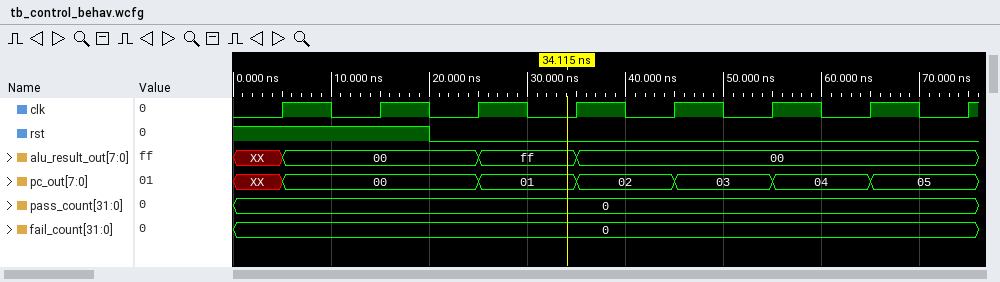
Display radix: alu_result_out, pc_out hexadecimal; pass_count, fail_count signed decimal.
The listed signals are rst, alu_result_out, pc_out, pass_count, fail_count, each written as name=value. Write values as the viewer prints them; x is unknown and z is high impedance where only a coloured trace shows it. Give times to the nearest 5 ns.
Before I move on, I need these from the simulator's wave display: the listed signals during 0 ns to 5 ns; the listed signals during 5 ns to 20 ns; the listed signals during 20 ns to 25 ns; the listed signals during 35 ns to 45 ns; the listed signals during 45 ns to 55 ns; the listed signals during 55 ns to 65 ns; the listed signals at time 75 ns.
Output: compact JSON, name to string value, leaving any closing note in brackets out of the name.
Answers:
{"the listed signals during 0 ns to 5 ns": "rst=1, alu_result_out=XX, pc_out=XX, pass_count=0, fail_count=0", "the listed signals during 5 ns to 20 ns": "rst=1, alu_result_out=00, pc_out=00, pass_count=0, fail_count=0", "the listed signals during 20 ns to 25 ns": "rst=0, alu_result_out=00, pc_out=00, pass_count=0, fail_count=0", "the listed signals during 35 ns to 45 ns": "rst=0, alu_result_out=00, pc_out=02, pass_count=0, fail_count=0", "the listed signals during 45 ns to 55 ns": "rst=0, alu_result_out=00, pc_out=03, pass_count=0, fail_count=0", "the listed signals during 55 ns to 65 ns": "rst=0, alu_result_out=00, pc_out=04, pass_count=0, fail_count=0", "the listed signals at time 75 ns": "rst=0, alu_result_out=00, pc_out=05, pass_count=0, fail_count=0"}
